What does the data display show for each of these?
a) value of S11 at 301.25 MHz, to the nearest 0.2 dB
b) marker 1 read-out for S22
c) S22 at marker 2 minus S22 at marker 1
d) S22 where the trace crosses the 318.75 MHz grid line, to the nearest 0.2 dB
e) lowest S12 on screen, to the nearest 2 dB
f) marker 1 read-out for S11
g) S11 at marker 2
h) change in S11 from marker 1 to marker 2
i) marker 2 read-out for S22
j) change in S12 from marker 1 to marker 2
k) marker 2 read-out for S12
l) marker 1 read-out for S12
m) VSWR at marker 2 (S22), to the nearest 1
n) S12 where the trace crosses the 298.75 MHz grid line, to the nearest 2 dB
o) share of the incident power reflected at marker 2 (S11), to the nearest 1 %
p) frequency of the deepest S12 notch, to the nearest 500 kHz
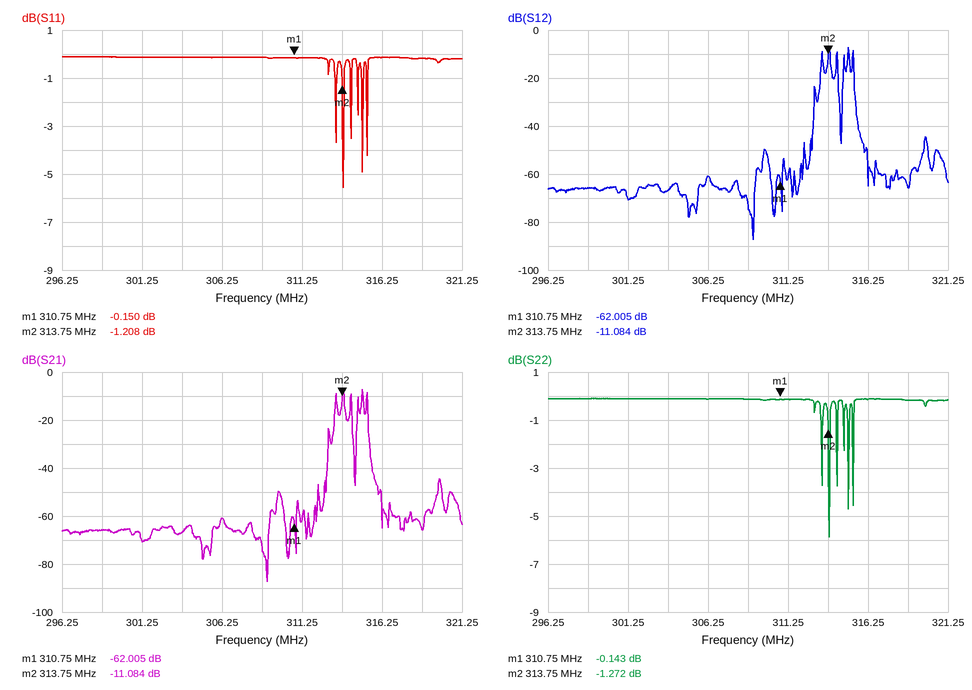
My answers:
-0.2 dB
-0.143 dB
-1.129 dB
-0.2 dB
-88 dB
-0.150 dB
-1.208 dB
-1.058 dB
-1.272 dB
50.921 dB
-11.084 dB
-62.005 dB
14
-66 dB
76 %
309.0 MHz
